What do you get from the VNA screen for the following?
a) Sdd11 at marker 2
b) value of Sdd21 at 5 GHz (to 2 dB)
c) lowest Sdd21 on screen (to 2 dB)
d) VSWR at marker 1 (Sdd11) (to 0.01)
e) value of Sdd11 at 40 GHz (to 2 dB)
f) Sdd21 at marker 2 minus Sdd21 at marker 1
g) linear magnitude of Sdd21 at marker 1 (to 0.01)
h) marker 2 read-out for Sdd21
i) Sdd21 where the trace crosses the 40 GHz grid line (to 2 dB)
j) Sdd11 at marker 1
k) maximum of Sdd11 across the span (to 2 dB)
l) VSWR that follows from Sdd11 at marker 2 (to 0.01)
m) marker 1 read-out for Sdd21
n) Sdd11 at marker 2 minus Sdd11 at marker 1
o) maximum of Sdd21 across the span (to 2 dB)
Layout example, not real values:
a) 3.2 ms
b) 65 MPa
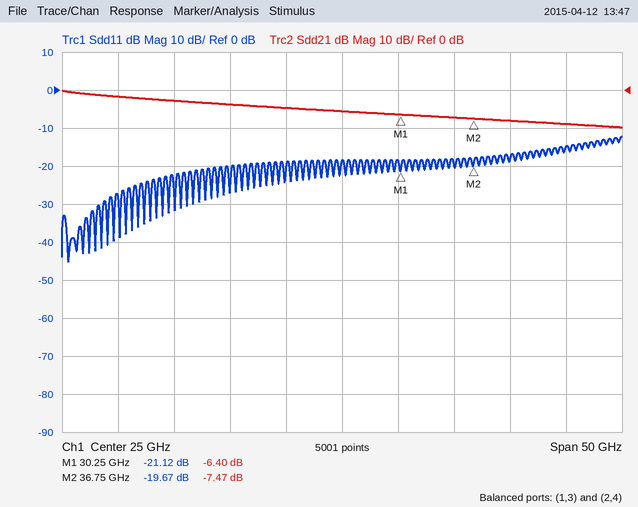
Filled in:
a) -19.67 dB
b) -2 dB
c) -10 dB
d) 1.19
e) -18 dB
f) -1.07 dB
g) 0.48
h) -7.47 dB
i) -8 dB
j) -21.12 dB
k) -12 dB
l) 1.23
m) -6.40 dB
n) 1.45 dB
o) 0 dB
